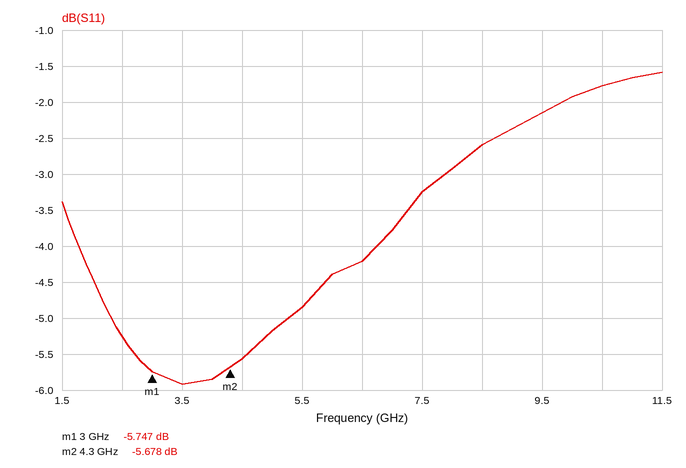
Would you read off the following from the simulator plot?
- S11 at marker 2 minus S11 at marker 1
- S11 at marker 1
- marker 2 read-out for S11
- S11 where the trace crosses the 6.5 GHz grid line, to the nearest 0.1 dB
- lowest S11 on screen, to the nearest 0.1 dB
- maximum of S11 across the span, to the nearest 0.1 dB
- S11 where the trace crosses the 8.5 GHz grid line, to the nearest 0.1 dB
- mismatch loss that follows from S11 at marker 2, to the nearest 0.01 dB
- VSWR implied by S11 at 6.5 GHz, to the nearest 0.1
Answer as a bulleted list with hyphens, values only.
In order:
- 0.069 dB
- -5.747 dB
- -5.678 dB
- -4.2 dB
- -5.9 dB
- -1.6 dB
- -2.6 dB
- 1.37 dB
- 4.2
